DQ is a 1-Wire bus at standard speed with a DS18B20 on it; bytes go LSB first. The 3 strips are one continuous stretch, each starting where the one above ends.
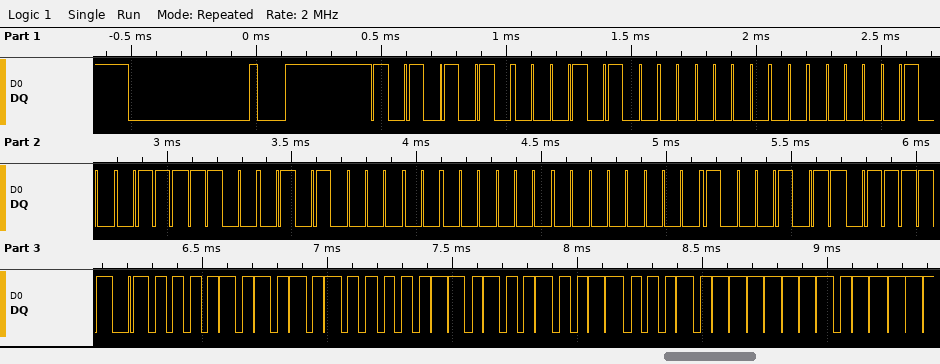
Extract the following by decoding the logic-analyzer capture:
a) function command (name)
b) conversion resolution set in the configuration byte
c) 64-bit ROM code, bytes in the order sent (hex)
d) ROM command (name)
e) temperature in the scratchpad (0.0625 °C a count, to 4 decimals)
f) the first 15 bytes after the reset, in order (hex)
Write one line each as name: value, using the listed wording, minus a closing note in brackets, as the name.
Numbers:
function command: Read Scratchpad
conversion resolution set in the configuration byte: 12 bits
64-bit ROM code, bytes in the order sent: 28 00 20 3E 0A 00 00 D1
ROM command: Match ROM
temperature in the scratchpad: 85.0000 °C
the first 15 bytes after the reset, in order: 55 28 00 20 3E 0A 00 00 D1 BE 50 05 4B 46 7F
